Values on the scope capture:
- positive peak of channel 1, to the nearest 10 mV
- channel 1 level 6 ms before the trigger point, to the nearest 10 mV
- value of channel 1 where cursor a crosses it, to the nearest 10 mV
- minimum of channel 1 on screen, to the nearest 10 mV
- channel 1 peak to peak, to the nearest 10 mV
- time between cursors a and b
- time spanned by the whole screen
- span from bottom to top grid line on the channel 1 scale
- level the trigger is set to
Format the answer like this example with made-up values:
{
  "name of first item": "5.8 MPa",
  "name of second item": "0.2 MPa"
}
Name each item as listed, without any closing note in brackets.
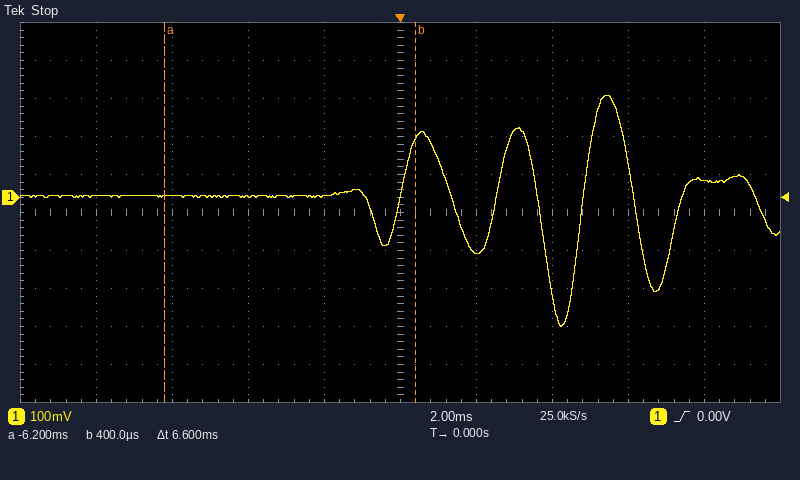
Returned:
{
  "positive peak of channel 1, to the nearest 10 mV": "270 mV",
  "channel 1 level 6 ms before the trigger point, to the nearest 10 mV": "0 mV",
  "value of channel 1 where cursor a crosses it, to the nearest 10 mV": "0 mV",
  "minimum of channel 1 on screen, to the nearest 10 mV": "-340 mV",
  "channel 1 peak to peak, to the nearest 10 mV": "610 mV",
  "time between cursors a and b": "6.6 ms",
  "time spanned by the whole screen": "20 ms",
  "span from bottom to top grid line on the channel 1 scale": "1 V",
  "level the trigger is set to": "0.00 V"
}
